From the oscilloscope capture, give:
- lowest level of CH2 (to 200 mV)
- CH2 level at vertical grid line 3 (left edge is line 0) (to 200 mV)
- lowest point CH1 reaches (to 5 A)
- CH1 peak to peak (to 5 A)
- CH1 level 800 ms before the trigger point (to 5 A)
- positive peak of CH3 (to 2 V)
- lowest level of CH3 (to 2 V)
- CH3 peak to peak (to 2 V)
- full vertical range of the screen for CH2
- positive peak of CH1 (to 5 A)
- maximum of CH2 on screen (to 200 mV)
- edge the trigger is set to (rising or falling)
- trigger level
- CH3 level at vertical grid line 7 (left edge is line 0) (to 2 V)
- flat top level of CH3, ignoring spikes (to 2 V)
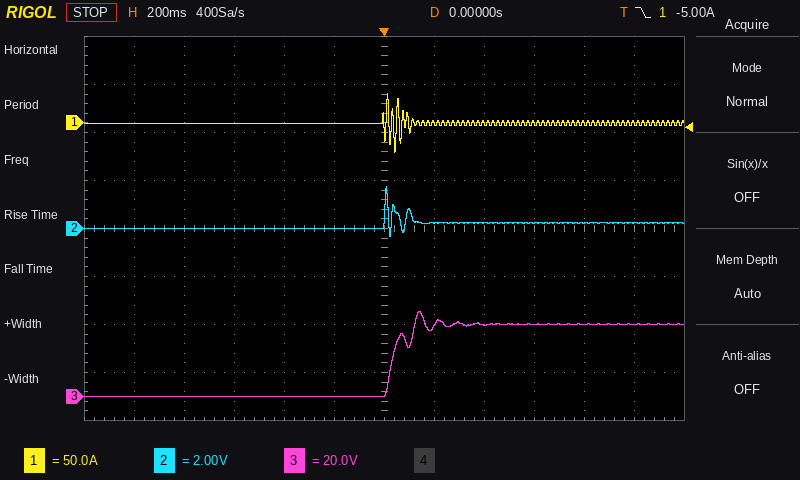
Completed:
-400 mV
0.0 V
-30 A
60 A
0 A
36 V
0 V
36 V
16 V
30 A
1.8 V
falling
-5.00 A
30 V
30 V
